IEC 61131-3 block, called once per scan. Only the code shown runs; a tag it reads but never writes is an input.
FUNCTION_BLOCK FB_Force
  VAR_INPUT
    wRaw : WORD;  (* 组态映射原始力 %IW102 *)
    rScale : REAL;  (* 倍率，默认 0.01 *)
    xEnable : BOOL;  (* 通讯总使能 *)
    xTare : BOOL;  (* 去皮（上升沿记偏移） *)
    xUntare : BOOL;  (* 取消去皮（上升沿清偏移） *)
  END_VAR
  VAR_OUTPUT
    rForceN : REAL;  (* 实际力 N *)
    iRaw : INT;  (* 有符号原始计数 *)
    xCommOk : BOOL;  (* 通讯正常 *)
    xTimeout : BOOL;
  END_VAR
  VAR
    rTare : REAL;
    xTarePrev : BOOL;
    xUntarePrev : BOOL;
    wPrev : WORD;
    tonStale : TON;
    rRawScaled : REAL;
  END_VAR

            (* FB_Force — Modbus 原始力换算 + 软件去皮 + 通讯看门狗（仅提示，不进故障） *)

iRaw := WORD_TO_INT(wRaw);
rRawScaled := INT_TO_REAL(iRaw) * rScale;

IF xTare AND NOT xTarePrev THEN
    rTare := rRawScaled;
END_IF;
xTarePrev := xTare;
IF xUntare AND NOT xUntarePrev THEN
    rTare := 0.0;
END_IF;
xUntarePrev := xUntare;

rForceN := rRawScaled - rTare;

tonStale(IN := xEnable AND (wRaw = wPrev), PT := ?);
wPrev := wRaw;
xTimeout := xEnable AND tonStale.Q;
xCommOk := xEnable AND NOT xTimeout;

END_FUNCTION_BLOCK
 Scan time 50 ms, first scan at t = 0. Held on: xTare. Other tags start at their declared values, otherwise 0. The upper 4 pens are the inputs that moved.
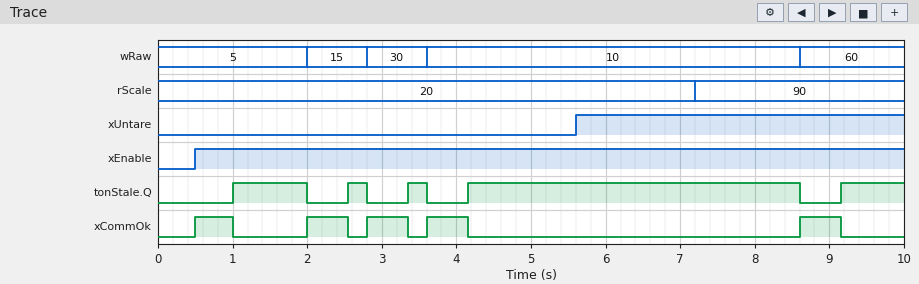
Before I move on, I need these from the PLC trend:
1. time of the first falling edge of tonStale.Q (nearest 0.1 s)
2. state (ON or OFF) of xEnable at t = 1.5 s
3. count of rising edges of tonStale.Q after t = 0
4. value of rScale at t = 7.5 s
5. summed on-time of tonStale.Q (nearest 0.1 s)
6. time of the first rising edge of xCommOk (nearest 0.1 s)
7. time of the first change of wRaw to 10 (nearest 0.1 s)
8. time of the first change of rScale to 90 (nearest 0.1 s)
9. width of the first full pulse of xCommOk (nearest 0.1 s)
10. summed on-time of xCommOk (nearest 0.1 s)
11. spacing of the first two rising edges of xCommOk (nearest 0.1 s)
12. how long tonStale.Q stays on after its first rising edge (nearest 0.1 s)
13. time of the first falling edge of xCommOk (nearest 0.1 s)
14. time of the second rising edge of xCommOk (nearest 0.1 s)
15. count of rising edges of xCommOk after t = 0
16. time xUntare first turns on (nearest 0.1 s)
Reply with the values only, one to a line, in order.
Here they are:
2.0 s
ON
5
90
6.8 s
0.5 s
3.6 s
7.2 s
0.5 s
2.7 s
1.5 s
1.0 s
1.0 s
2.0 s
5
5.6 s
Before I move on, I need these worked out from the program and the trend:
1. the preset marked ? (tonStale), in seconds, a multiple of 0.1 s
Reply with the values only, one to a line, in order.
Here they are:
0.5 s
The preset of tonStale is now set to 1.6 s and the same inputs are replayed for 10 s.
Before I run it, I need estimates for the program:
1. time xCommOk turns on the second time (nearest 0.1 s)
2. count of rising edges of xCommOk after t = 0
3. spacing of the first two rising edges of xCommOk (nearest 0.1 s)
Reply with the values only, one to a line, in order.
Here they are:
8.6 s
2
8.1 s
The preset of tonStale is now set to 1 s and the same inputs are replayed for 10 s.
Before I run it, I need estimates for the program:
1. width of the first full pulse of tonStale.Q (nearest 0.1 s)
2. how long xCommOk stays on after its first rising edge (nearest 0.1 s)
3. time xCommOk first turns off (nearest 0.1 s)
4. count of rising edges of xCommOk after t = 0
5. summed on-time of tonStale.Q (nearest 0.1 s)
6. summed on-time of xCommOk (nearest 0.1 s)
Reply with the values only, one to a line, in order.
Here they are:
0.5 s
1.0 s
1.5 s
3
4.8 s
4.7 s
